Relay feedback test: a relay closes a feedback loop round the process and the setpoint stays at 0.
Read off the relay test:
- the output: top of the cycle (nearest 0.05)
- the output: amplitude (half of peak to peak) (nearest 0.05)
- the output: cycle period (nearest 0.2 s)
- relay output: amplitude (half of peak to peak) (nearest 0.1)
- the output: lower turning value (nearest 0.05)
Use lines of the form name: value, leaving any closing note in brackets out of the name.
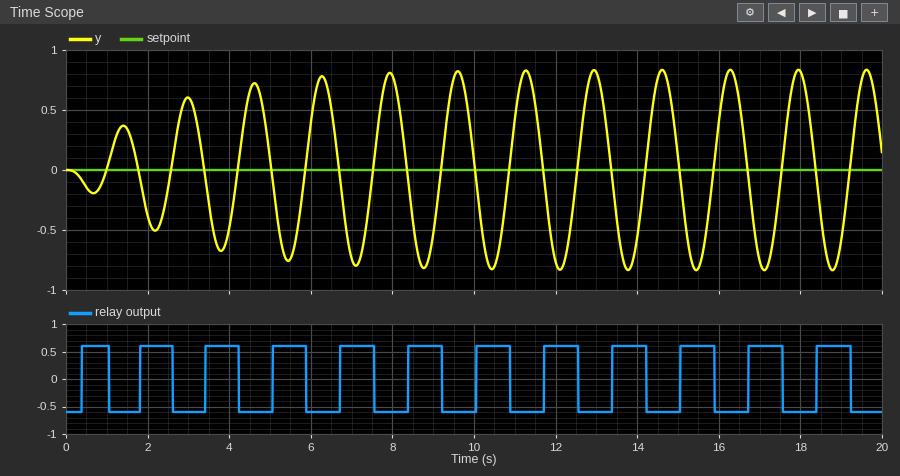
the output: top of the cycle: 0.85
the output: amplitude (half of peak to peak): 0.85
the output: cycle period: 1.6 s
relay output: amplitude (half of peak to peak): 0.6
the output: lower turning value: -0.85
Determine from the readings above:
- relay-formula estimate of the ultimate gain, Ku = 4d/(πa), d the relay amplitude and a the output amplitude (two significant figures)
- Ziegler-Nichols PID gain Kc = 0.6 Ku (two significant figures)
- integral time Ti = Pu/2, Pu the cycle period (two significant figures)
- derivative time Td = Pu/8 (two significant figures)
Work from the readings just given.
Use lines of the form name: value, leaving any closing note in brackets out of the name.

relay-formula estimate of the ultimate gain, Ku = 4d/(πa), d the relay amplitude and a the output amplitude: 0.90
Ziegler-Nichols PID gain Kc = 0.6 Ku: 0.54
integral time Ti = Pu/2, Pu the cycle period: 0.80 s
derivative time Td = Pu/8: 0.20 s
